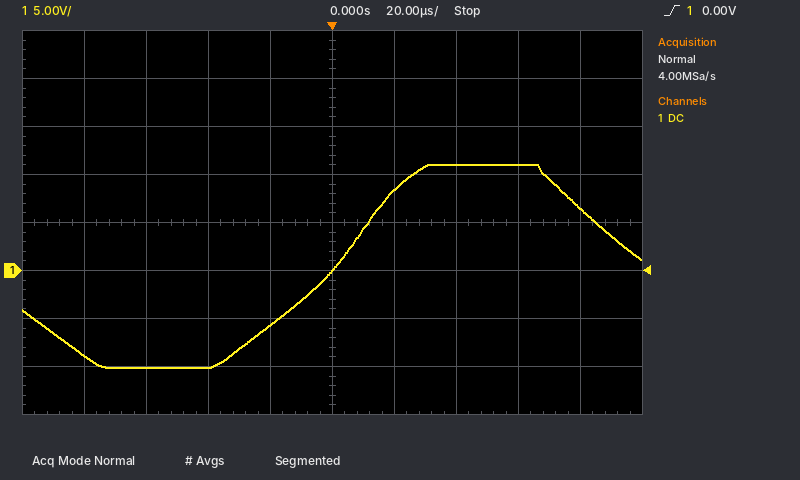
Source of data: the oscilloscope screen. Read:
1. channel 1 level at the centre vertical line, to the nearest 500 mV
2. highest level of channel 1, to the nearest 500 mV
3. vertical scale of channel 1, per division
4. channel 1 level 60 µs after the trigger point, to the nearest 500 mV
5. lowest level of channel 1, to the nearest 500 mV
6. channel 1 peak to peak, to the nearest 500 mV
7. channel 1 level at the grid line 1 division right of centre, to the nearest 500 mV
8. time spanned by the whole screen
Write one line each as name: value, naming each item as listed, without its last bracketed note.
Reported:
channel 1 level at the centre vertical line, to the nearest 500 mV: 0.0 V
highest level of channel 1, to the nearest 500 mV: 11.0 V
vertical scale of channel 1, per division: 5 V
channel 1 level 60 µs after the trigger point, to the nearest 500 mV: 11.0 V
lowest level of channel 1, to the nearest 500 mV: -10.0 V
channel 1 peak to peak, to the nearest 500 mV: 21.0 V
channel 1 level at the grid line 1 division right of centre, to the nearest 500 mV: 8.5 V
time spanned by the whole screen: 200 µs
